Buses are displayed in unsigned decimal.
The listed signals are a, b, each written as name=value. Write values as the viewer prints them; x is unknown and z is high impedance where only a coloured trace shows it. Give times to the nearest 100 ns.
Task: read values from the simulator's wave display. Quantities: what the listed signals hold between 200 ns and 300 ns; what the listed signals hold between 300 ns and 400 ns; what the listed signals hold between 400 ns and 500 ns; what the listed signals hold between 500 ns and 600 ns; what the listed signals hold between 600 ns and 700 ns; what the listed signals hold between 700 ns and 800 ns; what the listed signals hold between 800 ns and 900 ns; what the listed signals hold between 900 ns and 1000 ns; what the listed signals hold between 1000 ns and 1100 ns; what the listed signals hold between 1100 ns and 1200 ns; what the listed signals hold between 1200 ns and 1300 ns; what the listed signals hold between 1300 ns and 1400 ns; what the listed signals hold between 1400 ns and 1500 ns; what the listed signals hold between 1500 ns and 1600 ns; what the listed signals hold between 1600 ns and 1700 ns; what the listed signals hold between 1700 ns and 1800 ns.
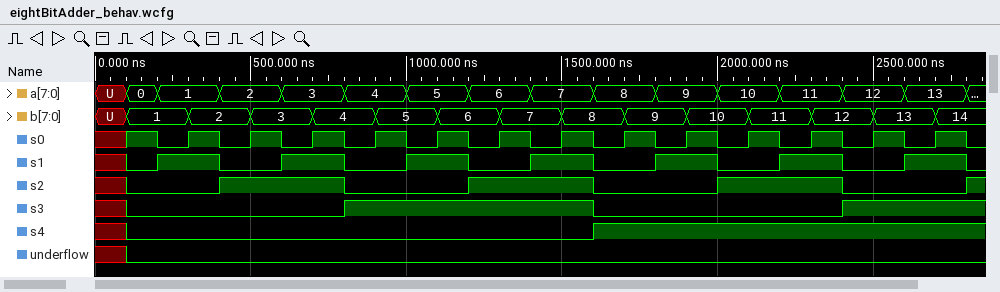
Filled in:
a=1, b=1
a=1, b=2
a=2, b=2
a=2, b=3
a=3, b=3
a=3, b=4
a=4, b=4
a=4, b=5
a=5, b=5
a=5, b=6
a=6, b=6
a=6, b=7
a=7, b=7
a=7, b=8
a=8, b=8
a=8, b=9
